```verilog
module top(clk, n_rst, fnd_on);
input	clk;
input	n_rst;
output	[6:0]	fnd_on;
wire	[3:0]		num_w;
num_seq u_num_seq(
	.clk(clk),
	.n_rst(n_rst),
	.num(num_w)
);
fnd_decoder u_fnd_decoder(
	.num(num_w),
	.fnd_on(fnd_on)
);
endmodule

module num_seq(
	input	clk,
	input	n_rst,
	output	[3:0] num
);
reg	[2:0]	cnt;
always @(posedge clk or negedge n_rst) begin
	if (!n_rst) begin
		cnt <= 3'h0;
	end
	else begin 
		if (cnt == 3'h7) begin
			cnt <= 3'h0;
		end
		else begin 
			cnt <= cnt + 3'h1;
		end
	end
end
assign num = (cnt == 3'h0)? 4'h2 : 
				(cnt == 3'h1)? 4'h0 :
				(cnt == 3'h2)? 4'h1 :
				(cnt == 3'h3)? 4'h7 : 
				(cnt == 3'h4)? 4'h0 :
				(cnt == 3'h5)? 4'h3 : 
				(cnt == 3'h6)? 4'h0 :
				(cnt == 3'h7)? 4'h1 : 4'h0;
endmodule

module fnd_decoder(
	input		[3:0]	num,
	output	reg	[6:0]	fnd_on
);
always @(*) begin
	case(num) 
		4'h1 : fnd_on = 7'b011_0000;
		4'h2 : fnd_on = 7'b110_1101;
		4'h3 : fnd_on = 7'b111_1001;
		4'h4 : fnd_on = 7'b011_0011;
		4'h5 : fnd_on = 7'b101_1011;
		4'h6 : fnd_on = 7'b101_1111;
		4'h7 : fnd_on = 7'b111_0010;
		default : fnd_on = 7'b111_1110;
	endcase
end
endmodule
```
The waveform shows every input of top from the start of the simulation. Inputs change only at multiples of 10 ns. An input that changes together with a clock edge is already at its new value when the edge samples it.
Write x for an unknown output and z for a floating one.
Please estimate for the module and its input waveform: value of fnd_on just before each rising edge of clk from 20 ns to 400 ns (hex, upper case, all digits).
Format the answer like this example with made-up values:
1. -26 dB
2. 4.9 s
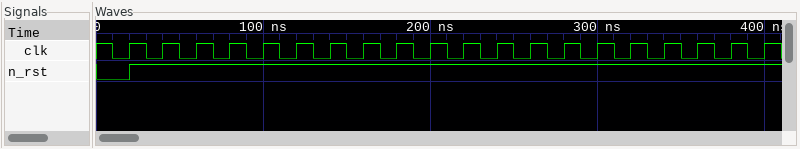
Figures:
1. 6D, 7E, 30, 72, 7E, 79, 7E, 30, 6D, 7E, 30, 72, 7E, 79, 7E, 30, 6D, 7E, 30, 72
